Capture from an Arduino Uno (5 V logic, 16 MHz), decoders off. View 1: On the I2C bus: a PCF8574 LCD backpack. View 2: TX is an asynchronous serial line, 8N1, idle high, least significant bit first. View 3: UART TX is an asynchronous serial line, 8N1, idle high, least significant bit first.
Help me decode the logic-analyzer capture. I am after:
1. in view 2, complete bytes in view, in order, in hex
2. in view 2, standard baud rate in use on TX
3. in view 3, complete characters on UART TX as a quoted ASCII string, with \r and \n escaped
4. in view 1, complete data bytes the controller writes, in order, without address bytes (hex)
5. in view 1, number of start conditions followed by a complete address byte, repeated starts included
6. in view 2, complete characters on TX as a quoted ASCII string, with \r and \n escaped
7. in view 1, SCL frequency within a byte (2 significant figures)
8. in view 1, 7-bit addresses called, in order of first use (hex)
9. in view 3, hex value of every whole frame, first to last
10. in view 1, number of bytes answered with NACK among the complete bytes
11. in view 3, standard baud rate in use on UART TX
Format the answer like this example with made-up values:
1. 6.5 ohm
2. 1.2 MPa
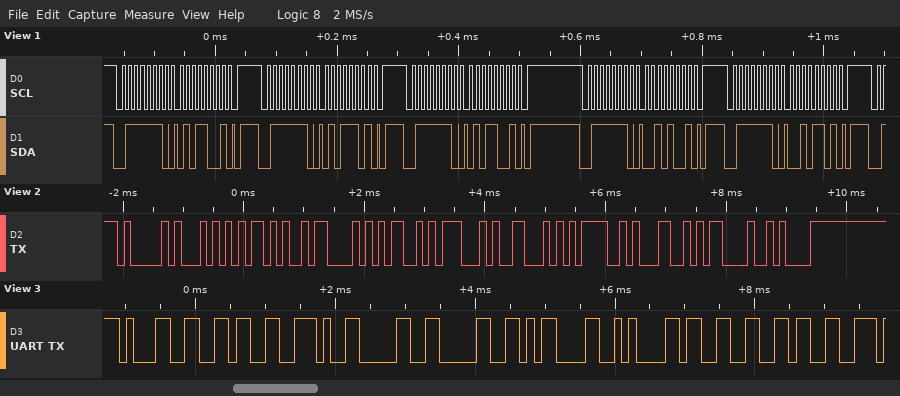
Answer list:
1. 0x41 0x54 0x2B 0x43 0x4D 0x47 0x46 0x3D 0x31 0x0D 0x0A
2. 9600 baud
3. "16.00\r\n36"
4. 59 5D 59 29 2D
5. 5
6. "AT+CMGF=1\r\n"
7. 100 kHz
8. 0x3F
9. 0x31 0x36 0x2E 0x30 0x30 0x0D 0x0A 0x33 0x36
10. 0
11. 9600 baud
